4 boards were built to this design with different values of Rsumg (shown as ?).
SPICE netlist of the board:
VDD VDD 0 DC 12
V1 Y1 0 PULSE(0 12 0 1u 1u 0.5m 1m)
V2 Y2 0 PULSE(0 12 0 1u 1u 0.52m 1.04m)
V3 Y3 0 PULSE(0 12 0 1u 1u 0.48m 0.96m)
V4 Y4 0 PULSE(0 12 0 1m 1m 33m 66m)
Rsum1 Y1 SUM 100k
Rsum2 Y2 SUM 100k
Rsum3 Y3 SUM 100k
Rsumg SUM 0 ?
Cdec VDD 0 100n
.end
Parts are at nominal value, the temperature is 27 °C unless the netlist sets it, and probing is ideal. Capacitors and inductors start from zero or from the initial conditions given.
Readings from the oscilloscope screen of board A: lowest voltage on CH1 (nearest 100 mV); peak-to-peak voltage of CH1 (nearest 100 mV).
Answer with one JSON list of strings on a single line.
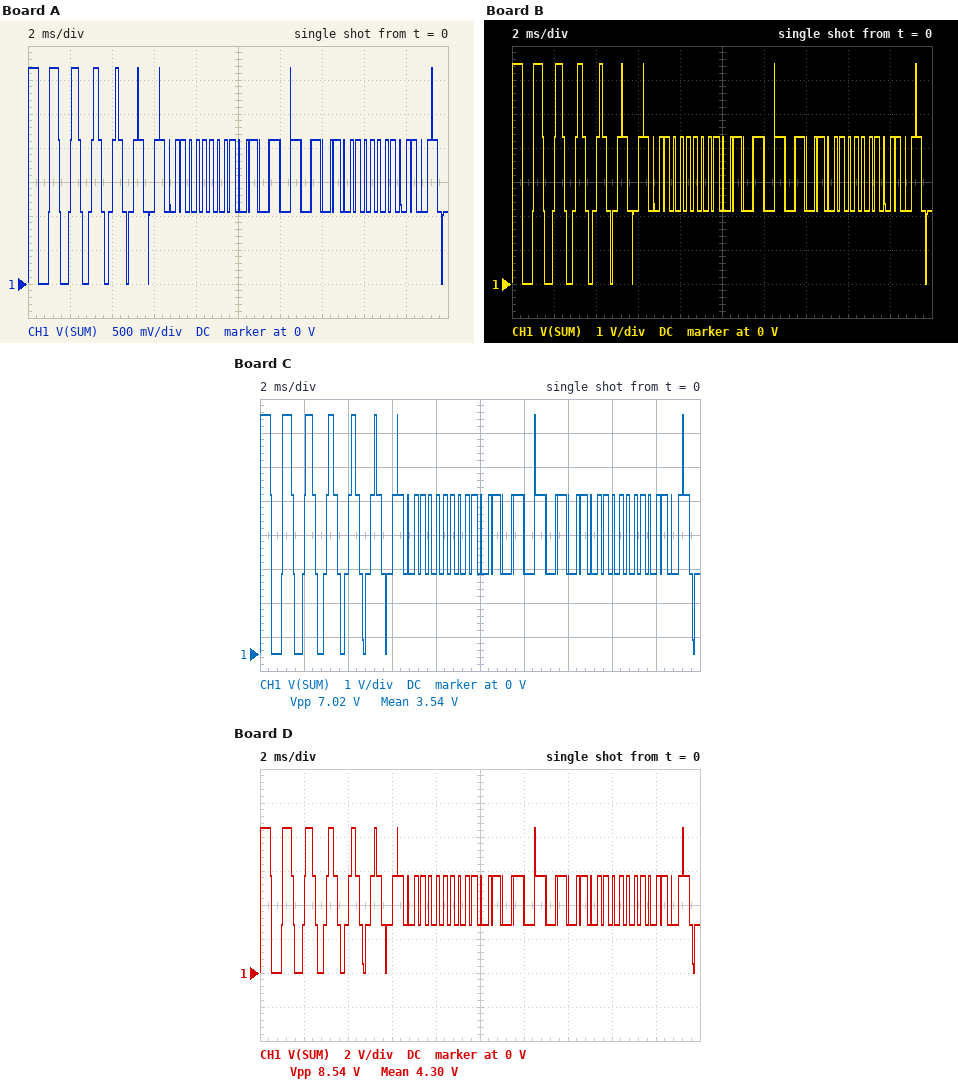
["0 V", "3.2 V"]
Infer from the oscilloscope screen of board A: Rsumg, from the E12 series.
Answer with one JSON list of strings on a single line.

["12 kΩ"]
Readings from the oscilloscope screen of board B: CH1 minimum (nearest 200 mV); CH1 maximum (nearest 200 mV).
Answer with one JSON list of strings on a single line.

["0 V", "6.4 V"]
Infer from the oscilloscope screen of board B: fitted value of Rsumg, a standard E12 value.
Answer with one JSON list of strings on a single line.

["39 kΩ"]
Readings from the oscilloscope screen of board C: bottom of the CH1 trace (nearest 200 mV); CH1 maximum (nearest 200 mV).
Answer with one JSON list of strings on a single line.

["0 V", "7.0 V"]
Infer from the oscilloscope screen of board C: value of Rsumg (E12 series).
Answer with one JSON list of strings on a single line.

["47 kΩ"]
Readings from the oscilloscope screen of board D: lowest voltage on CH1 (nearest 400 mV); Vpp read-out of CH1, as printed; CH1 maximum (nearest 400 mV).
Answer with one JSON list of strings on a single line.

["0 V", "8.54 V", "8.4 V"]
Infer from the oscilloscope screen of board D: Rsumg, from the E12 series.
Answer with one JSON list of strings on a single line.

["82 kΩ"]
